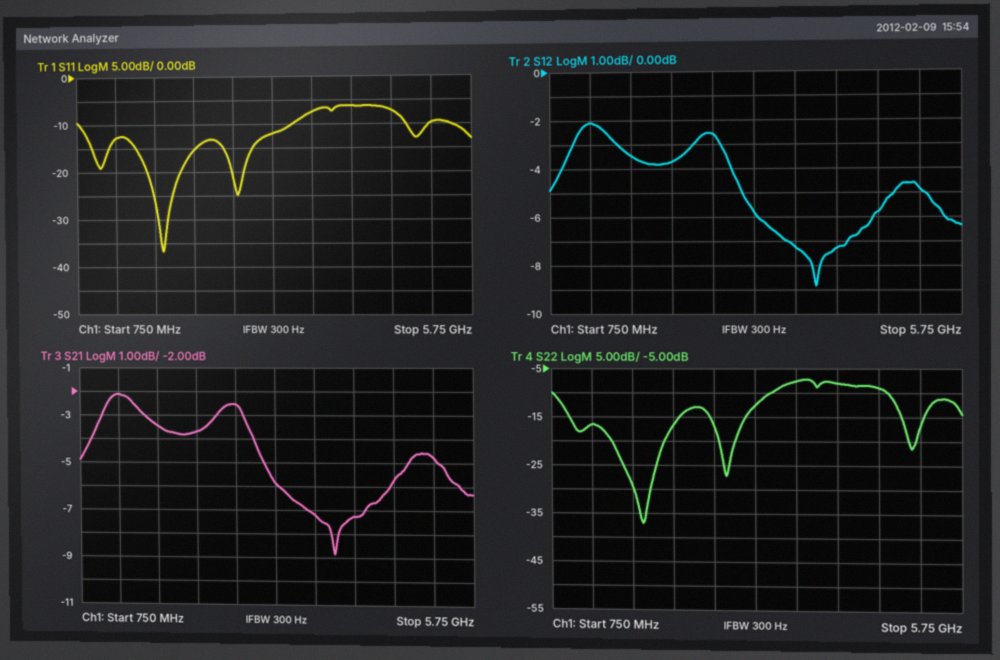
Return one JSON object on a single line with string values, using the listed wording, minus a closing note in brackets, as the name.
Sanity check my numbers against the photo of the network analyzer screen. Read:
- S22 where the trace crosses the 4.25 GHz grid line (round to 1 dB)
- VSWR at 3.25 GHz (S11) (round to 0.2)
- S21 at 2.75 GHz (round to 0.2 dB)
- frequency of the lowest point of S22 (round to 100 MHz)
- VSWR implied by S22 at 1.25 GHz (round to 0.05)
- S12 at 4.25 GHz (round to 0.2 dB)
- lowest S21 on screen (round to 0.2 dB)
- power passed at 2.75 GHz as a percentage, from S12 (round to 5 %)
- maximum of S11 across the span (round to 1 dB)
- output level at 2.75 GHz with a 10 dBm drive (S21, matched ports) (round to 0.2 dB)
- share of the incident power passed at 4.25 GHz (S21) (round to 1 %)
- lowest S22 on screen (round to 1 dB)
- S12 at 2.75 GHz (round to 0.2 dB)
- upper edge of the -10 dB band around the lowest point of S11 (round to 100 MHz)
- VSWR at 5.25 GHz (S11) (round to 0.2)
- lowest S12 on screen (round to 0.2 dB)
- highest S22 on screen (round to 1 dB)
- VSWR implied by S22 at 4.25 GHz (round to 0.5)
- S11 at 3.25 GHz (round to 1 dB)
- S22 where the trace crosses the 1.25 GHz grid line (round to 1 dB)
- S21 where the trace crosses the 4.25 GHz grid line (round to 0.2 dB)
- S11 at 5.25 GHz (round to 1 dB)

{"S22 where the trace crosses the 4.25 GHz grid line": "-8 dB", "VSWR at 3.25 GHz (S11)": "1.6", "S21 at 2.75 GHz": "-2.6 dB", "frequency of the lowest point of S22": "1.9 GHz", "VSWR implied by S22 at 1.25 GHz": "1.35", "S12 at 4.25 GHz": "-7.2 dB", "lowest S21 on screen": "-8.8 dB", "power passed at 2.75 GHz as a percentage, from S12": "55 %", "maximum of S11 across the span": "-6 dB", "output level at 2.75 GHz with a 10 dBm drive (S21, matched ports)": "7.4 dBm", "share of the incident power passed at 4.25 GHz (S21)": "19 %", "lowest S22 on screen": "-37 dB", "S12 at 2.75 GHz": "-2.6 dB", "upper edge of the -10 dB band around the lowest point of S11": "3.5 GHz", "VSWR at 5.25 GHz (S11)": "2.0", "lowest S12 on screen": "-8.8 dB", "highest S22 on screen": "-7 dB", "VSWR implied by S22 at 4.25 GHz": "2.5", "S11 at 3.25 GHz": "-12 dB", "S22 where the trace crosses the 1.25 GHz grid line": "-17 dB", "S21 where the trace crosses the 4.25 GHz grid line": "-7.2 dB", "S11 at 5.25 GHz": "-10 dB"}
